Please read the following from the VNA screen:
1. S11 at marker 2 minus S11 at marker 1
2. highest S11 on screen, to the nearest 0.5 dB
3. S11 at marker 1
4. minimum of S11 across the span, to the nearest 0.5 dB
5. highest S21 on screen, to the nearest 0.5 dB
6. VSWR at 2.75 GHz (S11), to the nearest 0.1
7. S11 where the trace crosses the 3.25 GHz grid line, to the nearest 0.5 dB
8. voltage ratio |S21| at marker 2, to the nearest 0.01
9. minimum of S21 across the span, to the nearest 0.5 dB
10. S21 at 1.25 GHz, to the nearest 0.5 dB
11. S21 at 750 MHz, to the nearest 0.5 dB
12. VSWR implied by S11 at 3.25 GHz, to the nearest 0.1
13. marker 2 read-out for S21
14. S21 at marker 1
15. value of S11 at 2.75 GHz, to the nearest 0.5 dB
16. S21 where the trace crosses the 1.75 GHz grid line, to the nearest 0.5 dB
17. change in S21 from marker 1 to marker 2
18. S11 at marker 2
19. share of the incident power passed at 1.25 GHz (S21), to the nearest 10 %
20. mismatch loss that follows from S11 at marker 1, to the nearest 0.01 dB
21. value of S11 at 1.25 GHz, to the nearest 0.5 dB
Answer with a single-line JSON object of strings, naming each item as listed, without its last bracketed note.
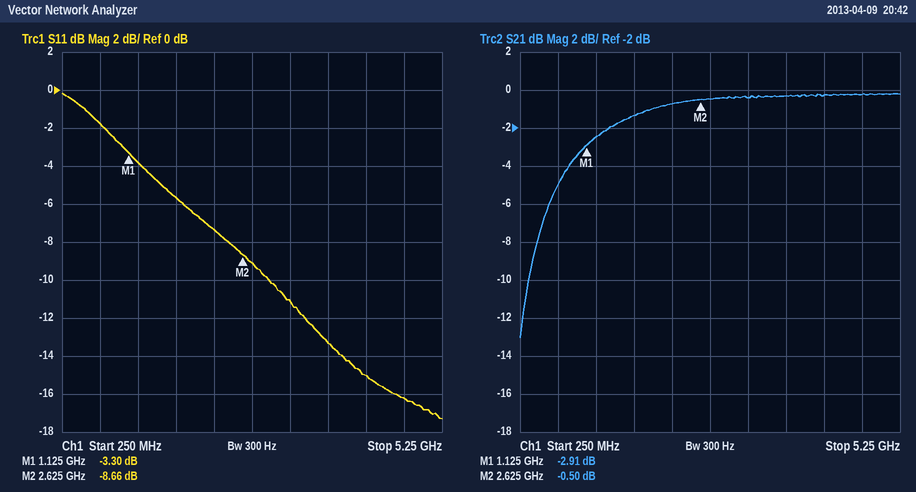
{"S11 at marker 2 minus S11 at marker 1": "-5.36 dB", "highest S11 on screen, to the nearest 0.5 dB": "0.0 dB", "S11 at marker 1": "-3.30 dB", "minimum of S11 across the span, to the nearest 0.5 dB": "-17.5 dB", "highest S21 on screen, to the nearest 0.5 dB": "0.0 dB", "VSWR at 2.75 GHz (S11), to the nearest 0.1": "2.1", "S11 where the trace crosses the 3.25 GHz grid line, to the nearest 0.5 dB": "-11.0 dB", "voltage ratio |S21| at marker 2, to the nearest 0.01": "0.94", "minimum of S21 across the span, to the nearest 0.5 dB": "-13.0 dB", "S21 at 1.25 GHz, to the nearest 0.5 dB": "-2.5 dB", "S21 at 750 MHz, to the nearest 0.5 dB": "-5.0 dB", "VSWR implied by S11 at 3.25 GHz, to the nearest 0.1": "1.8", "marker 2 read-out for S21": "-0.50 dB", "S21 at marker 1": "-2.91 dB", "value of S11 at 2.75 GHz, to the nearest 0.5 dB": "-9.0 dB", "S21 where the trace crosses the 1.75 GHz grid line, to the nearest 0.5 dB": "-1.5 dB", "change in S21 from marker 1 to marker 2": "2.41 dB", "S11 at marker 2": "-8.66 dB", "share of the incident power passed at 1.25 GHz (S21), to the nearest 10 %": "60 %", "mismatch loss that follows from S11 at marker 1, to the nearest 0.01 dB": "2.74 dB", "value of S11 at 1.25 GHz, to the nearest 0.5 dB": "-4.0 dB"}
